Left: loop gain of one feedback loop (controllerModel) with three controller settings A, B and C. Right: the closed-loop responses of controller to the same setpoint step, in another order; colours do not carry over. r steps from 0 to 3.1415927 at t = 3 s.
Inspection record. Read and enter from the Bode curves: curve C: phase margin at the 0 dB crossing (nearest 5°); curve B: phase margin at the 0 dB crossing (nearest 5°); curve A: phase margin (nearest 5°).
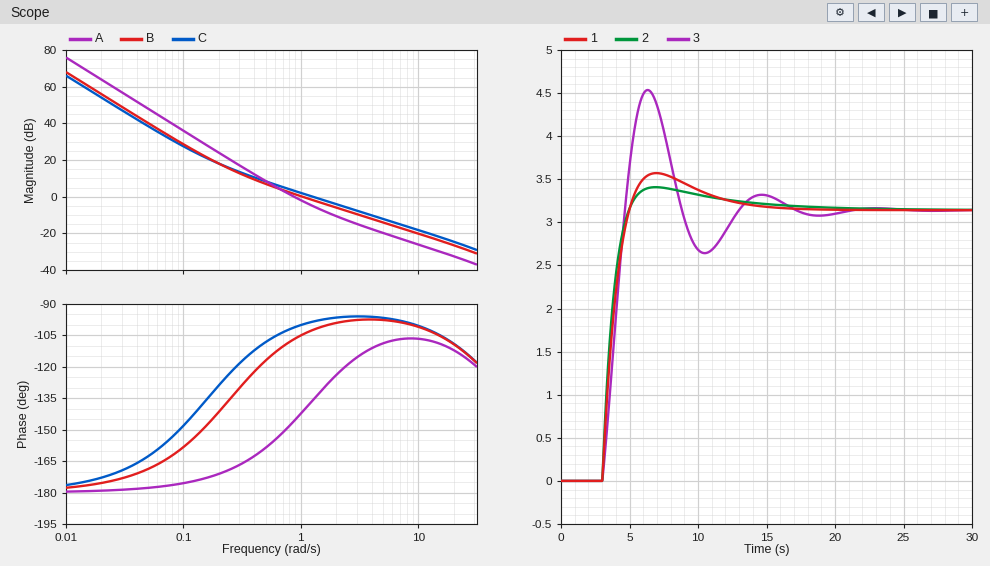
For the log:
80°
75°
35°
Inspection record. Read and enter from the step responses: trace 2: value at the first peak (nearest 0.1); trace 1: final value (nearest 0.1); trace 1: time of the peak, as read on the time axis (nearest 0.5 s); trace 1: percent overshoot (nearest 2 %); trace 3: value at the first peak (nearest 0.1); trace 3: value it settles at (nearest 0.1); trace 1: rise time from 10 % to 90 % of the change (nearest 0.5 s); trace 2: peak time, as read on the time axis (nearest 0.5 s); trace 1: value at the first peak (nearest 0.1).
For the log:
3.4
3.1
7.0 s
14 %
4.5
3.1
1.5 s
7.0 s
3.6
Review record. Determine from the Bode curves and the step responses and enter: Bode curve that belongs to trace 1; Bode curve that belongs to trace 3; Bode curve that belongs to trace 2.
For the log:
B
A
C
